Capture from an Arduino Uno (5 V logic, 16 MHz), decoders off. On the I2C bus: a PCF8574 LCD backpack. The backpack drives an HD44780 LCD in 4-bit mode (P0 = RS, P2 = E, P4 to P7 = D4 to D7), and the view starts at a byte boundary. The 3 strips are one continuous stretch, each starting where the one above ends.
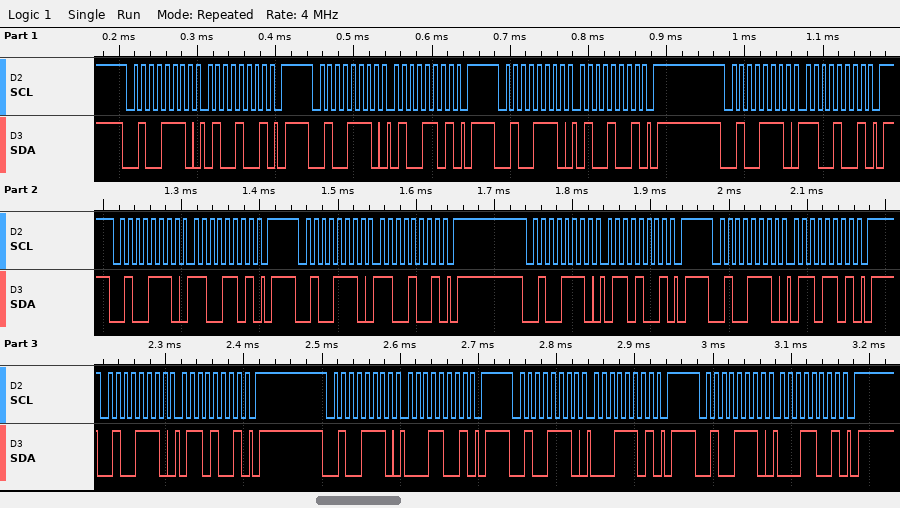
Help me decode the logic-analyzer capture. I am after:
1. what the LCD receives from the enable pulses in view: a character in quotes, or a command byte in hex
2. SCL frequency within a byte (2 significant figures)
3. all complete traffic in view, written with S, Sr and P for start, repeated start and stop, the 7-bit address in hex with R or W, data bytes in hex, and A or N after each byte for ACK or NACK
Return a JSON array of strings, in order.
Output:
["'L' 'a'", "100 kHz", "S 27W A 49 A P S 27W A 4D A P S 27W A 49 A P S 27W A C9 A P S 27W A CD A P S 27W A C9 A P S 27W A 69 A P S 27W A 6D A P S 27W A 69 A P S 27W A 19 A P S 27W A 1D A P S 27W A 19 A P"]
